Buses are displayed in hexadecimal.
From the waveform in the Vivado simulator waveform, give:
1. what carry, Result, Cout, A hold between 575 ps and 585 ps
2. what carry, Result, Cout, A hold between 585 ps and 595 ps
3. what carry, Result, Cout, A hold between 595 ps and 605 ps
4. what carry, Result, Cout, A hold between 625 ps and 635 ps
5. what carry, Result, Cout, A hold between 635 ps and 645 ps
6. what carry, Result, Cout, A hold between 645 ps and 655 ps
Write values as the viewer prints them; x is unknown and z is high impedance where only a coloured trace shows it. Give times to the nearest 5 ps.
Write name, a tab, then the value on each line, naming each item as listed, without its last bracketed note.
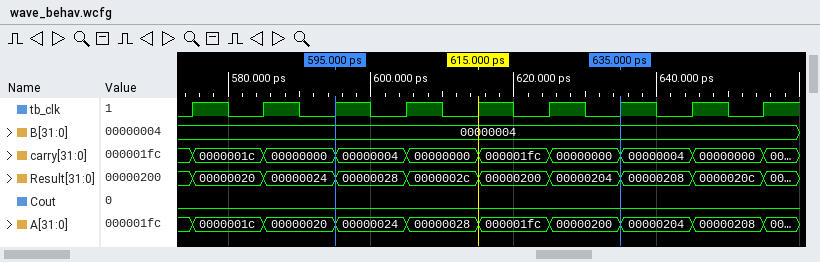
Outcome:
what carry, Result, Cout, A hold between 575 ps and 585 ps	carry=0000001c, Result=00000020, Cout=0, A=0000001c
what carry, Result, Cout, A hold between 585 ps and 595 ps	carry=00000000, Result=00000024, Cout=0, A=00000020
what carry, Result, Cout, A hold between 595 ps and 605 ps	carry=00000004, Result=00000028, Cout=0, A=00000024
what carry, Result, Cout, A hold between 625 ps and 635 ps	carry=00000000, Result=00000204, Cout=0, A=00000200
what carry, Result, Cout, A hold between 635 ps and 645 ps	carry=00000004, Result=00000208, Cout=0, A=00000204
what carry, Result, Cout, A hold between 645 ps and 655 ps	carry=00000000, Result=0000020c, Cout=0, A=00000208
